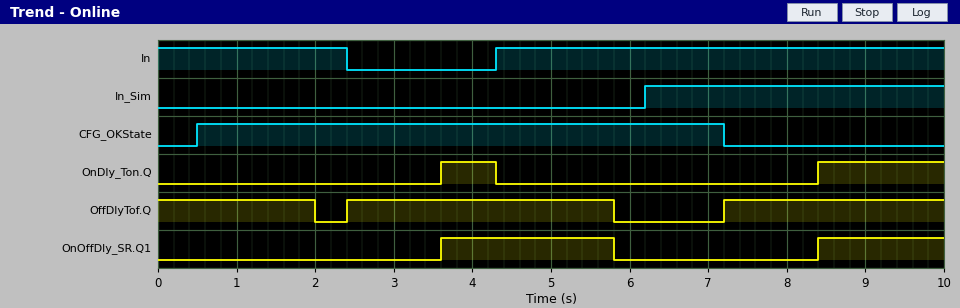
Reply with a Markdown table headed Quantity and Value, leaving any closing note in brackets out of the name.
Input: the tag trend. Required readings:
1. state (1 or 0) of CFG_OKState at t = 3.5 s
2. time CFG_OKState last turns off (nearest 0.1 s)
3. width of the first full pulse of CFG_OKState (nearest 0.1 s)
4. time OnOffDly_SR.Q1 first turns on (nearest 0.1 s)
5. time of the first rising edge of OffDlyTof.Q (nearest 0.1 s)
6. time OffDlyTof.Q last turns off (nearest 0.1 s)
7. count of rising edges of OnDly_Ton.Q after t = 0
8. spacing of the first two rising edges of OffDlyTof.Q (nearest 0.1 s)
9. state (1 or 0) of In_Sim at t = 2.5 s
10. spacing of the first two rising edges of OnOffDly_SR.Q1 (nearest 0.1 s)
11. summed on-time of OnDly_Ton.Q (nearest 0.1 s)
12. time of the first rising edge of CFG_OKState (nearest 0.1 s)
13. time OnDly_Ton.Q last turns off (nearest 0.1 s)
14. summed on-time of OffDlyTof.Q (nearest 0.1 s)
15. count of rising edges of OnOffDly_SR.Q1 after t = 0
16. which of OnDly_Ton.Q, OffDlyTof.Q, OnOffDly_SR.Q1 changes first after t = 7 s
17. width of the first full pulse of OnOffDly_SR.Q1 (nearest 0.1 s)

| Quantity | Value |
|---|---|
| state (1 or 0) of CFG_OKState at t = 3.5 s | 1 |
| time CFG_OKState last turns off | 7.2 s |
| width of the first full pulse of CFG_OKState | 6.7 s |
| time OnOffDly_SR.Q1 first turns on | 3.6 s |
| time of the first rising edge of OffDlyTof.Q | 2.4 s |
| time OffDlyTof.Q last turns off | 5.8 s |
| count of rising edges of OnDly_Ton.Q after t = 0 | 2 |
| spacing of the first two rising edges of OffDlyTof.Q | 4.8 s |
| state (1 or 0) of In_Sim at t = 2.5 s | 0 |
| spacing of the first two rising edges of OnOffDly_SR.Q1 | 4.8 s |
| summed on-time of OnDly_Ton.Q | 2.3 s |
| time of the first rising edge of CFG_OKState | 0.5 s |
| time OnDly_Ton.Q last turns off | 4.3 s |
| summed on-time of OffDlyTof.Q | 8.2 s |
| count of rising edges of OnOffDly_SR.Q1 after t = 0 | 2 |
| which of OnDly_Ton.Q, OffDlyTof.Q, OnOffDly_SR.Q1 changes first after t = 7 s | OffDlyTof.Q |
| width of the first full pulse of OnOffDly_SR.Q1 | 2.2 s |
